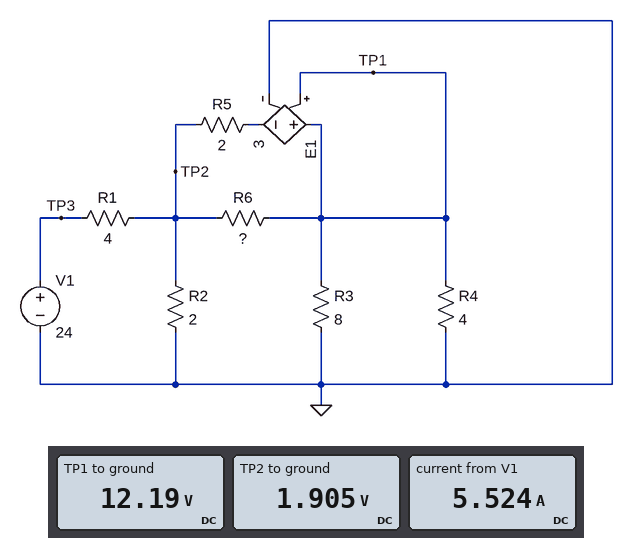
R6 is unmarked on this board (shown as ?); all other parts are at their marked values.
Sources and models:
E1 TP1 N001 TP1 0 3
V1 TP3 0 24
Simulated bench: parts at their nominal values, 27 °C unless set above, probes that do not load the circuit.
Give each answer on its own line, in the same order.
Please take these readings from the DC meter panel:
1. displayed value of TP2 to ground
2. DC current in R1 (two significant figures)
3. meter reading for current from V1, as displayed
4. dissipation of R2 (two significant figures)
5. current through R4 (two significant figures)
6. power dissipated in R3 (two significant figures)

1.905 V
5.5 A
5.524 A
1.8 W
3.0 A
19 W
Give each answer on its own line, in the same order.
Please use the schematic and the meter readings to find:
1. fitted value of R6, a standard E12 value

1.2 Ω
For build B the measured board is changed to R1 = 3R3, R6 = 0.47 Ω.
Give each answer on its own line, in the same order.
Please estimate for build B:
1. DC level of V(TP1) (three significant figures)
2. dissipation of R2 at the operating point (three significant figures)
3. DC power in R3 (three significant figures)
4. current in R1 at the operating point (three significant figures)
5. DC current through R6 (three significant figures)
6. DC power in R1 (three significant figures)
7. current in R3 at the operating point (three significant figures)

8.72 V
12.4 W
9.50 W
5.76 A
7.94 A
110 W
1.09 A
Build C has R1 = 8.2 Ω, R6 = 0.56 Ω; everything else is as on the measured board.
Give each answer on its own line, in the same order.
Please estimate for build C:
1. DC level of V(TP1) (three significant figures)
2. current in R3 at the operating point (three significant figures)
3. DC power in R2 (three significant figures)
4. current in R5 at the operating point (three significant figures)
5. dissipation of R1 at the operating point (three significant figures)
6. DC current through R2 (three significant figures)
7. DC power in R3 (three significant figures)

4.24 V
530 mA
2.31 W
5.31 A
58.2 W
1.08 A
2.24 W
